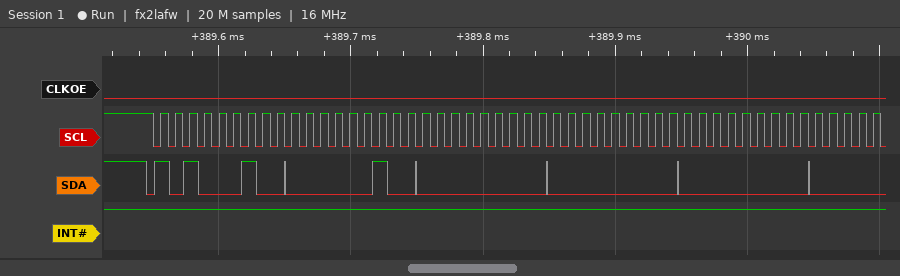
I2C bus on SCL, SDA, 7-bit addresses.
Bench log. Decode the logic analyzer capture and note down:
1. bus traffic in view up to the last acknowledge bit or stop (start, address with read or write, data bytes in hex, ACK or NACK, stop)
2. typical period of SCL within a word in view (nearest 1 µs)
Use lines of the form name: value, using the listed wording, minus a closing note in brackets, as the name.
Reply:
bus traffic in view up to the last acknowledge bit or stop: start, address 51 write ACK, 02 ACK, 00 ACK, 00 ACK, 00 ACK
typical period of SCL within a word in view: 11 µs
